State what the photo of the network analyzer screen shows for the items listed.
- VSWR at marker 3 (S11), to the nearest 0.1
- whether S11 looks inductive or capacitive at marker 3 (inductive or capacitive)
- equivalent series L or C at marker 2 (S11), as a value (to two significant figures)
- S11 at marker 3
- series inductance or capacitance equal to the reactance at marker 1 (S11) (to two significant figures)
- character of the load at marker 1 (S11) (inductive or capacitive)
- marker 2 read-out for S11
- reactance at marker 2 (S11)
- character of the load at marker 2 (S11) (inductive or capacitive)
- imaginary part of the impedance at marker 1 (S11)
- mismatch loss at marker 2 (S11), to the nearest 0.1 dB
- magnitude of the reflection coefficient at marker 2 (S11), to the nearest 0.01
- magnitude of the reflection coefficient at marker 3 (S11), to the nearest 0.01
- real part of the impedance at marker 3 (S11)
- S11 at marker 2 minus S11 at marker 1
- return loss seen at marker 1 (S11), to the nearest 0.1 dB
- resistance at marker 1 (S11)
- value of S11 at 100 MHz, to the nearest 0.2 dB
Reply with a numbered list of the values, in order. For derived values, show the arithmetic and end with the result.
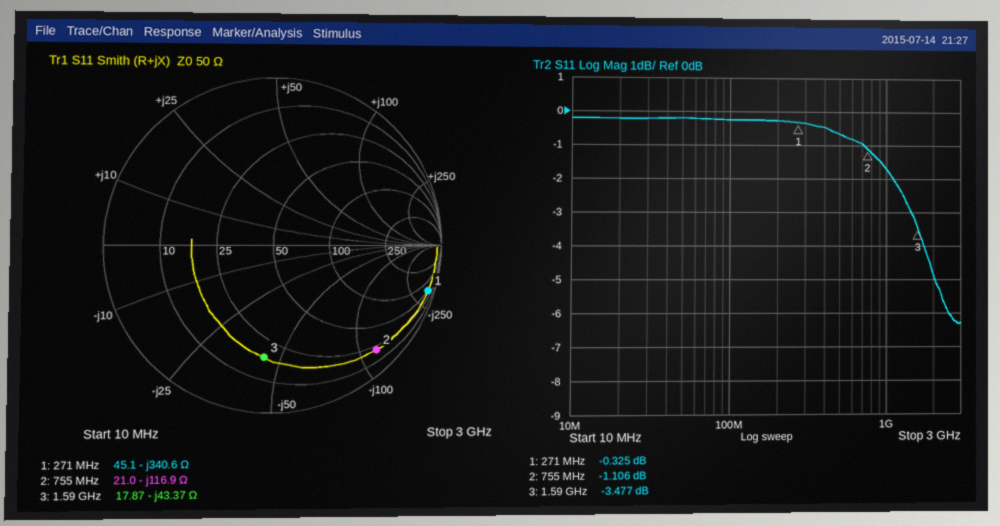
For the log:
1. 5.1
2. capacitive
3. C = 1/(2π × 755 MHz × 116.9 Ω) ≈ 1.8 pF
4. -3.477 dB
5. C = 1/(2π × 271 MHz × 340.6 Ω) ≈ 1.7 pF
6. capacitive
7. -1.106 dB
8. -116.9 Ω
9. capacitive
10. -340.6 Ω
11. −10 log10(1 − 10^(-1.106/10)) ≈ 6.5 dB
12. 0.88
13. 10^(-3.477/20) ≈ 0.67
14. 17.87 Ω
15. -1.106 − (-0.325) = -0.781 dB
16. 0.3 dB
17. 45.1 Ω
18. -0.2 dB
